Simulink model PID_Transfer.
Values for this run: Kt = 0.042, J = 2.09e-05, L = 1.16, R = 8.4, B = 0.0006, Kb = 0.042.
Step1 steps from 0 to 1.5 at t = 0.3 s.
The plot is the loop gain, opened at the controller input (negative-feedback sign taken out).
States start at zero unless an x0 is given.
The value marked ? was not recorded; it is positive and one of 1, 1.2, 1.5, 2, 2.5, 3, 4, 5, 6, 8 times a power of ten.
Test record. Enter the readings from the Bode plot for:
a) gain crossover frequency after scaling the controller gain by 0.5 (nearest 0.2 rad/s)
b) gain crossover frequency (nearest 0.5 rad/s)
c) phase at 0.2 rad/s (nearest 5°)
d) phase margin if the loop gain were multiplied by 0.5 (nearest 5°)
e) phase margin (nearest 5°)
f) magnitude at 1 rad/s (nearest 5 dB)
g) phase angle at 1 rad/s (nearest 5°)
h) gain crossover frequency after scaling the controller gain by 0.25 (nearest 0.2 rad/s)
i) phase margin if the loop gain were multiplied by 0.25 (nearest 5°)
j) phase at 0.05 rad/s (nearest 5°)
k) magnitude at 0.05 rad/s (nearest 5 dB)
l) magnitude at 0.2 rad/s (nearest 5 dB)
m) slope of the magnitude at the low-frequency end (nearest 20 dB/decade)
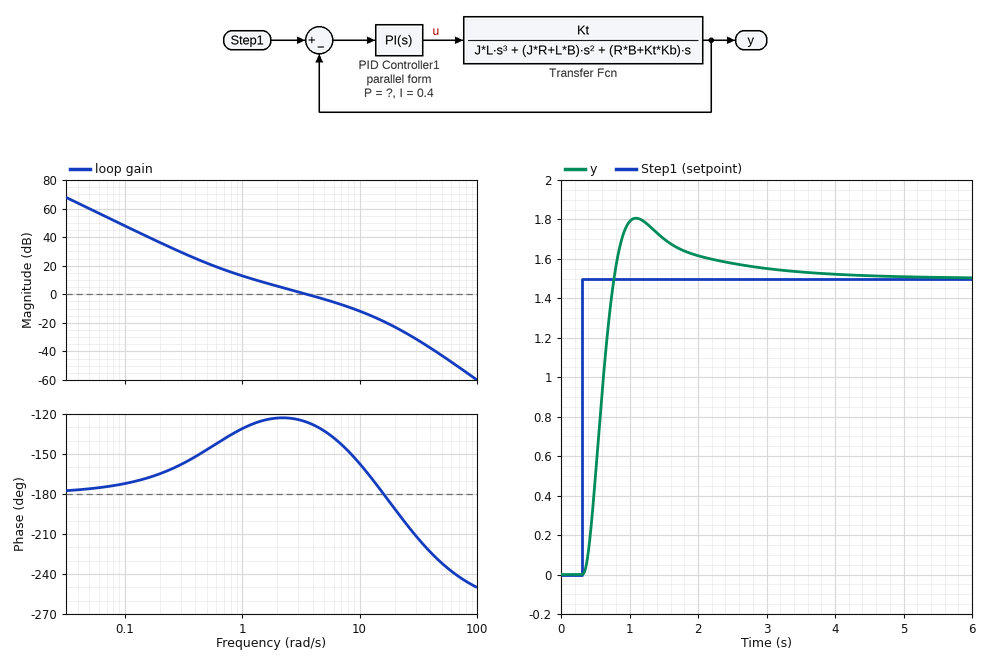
2.0 rad/s
3.5 rad/s
-165°
55°
55°
15 dB
-130°
1.0 rad/s
50°
-175°
60 dB
35 dB
-40 dB/decade
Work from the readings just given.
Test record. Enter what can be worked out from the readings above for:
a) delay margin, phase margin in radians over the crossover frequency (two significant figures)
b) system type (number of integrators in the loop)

0.27 s
2
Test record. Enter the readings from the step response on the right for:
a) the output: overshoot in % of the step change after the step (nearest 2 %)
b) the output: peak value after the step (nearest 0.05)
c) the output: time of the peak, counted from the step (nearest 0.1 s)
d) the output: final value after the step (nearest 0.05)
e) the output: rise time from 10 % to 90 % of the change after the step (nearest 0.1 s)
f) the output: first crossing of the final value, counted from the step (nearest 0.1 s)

20 %
1.80
0.8 s
1.50
0.3 s
0.5 s
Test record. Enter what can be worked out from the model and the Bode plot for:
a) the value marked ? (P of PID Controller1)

0.6
